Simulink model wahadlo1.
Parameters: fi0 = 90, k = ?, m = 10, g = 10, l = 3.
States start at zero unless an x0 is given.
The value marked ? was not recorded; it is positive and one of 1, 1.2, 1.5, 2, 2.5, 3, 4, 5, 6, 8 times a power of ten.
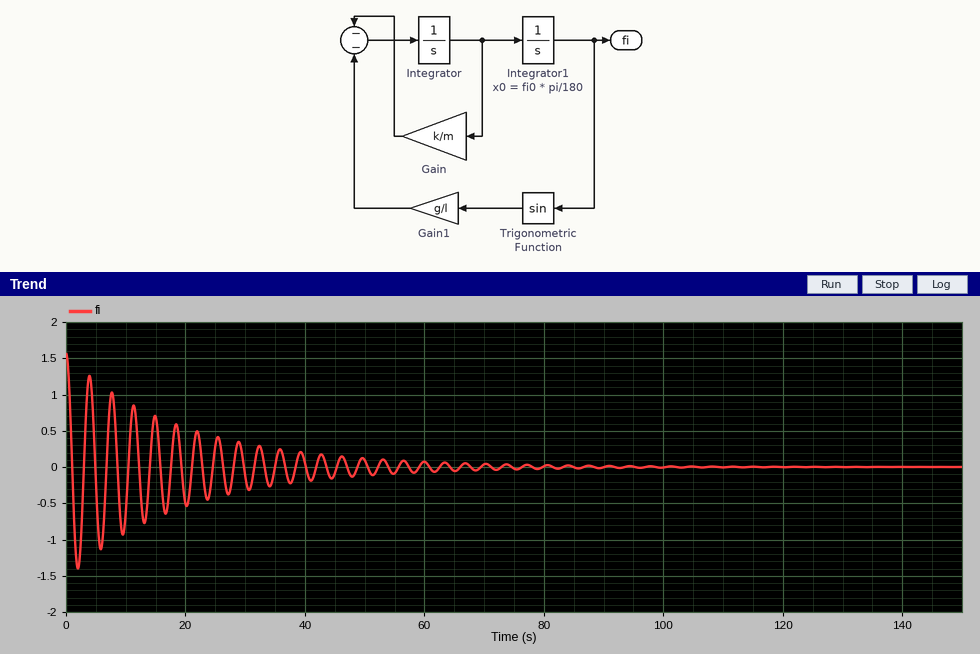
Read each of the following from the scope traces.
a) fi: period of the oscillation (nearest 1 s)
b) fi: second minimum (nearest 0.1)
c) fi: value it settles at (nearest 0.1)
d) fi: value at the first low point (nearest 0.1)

4 s
-1.1
0.0
-1.4
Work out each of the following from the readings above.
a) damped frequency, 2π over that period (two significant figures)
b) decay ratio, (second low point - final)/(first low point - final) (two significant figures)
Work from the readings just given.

1.6 rad/s
0.79
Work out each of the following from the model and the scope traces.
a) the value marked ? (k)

1
